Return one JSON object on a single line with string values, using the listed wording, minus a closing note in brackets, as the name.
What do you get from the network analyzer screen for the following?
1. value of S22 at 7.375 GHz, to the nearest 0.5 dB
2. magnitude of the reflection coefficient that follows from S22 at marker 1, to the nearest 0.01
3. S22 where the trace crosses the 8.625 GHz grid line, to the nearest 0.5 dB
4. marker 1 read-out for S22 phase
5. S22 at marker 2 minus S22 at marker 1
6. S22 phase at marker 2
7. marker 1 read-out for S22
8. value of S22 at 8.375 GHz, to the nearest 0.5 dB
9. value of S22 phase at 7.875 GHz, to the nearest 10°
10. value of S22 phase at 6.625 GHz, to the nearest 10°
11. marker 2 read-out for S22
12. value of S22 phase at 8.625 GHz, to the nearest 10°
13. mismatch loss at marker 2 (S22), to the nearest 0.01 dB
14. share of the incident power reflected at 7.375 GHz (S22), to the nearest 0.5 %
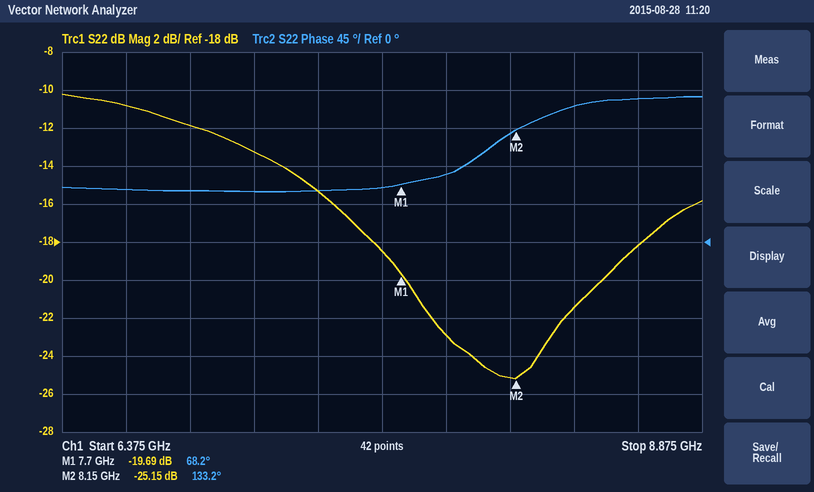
{"value of S22 at 7.375 GHz, to the nearest 0.5 dB": "-15.5 dB", "magnitude of the reflection coefficient that follows from S22 at marker 1, to the nearest 0.01": "0.10", "S22 where the trace crosses the 8.625 GHz grid line, to the nearest 0.5 dB": "-18.0 dB", "marker 1 read-out for S22 phase": "68.2°", "S22 at marker 2 minus S22 at marker 1": "-5.46 dB", "S22 phase at marker 2": "133.2°", "marker 1 read-out for S22": "-19.69 dB", "value of S22 at 8.375 GHz, to the nearest 0.5 dB": "-21.5 dB", "value of S22 phase at 7.875 GHz, to the nearest 10°": "80°", "value of S22 phase at 6.625 GHz, to the nearest 10°": "60°", "marker 2 read-out for S22": "-25.15 dB", "value of S22 phase at 8.625 GHz, to the nearest 10°": "170°", "mismatch loss at marker 2 (S22), to the nearest 0.01 dB": "0.01 dB", "share of the incident power reflected at 7.375 GHz (S22), to the nearest 0.5 %": "3.0 %"}
